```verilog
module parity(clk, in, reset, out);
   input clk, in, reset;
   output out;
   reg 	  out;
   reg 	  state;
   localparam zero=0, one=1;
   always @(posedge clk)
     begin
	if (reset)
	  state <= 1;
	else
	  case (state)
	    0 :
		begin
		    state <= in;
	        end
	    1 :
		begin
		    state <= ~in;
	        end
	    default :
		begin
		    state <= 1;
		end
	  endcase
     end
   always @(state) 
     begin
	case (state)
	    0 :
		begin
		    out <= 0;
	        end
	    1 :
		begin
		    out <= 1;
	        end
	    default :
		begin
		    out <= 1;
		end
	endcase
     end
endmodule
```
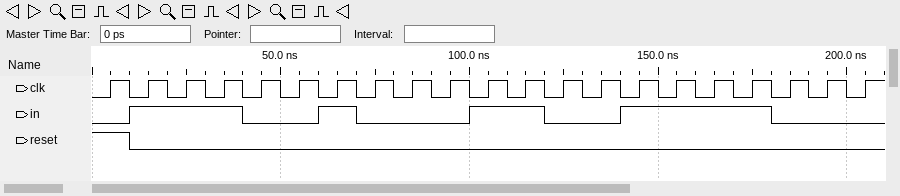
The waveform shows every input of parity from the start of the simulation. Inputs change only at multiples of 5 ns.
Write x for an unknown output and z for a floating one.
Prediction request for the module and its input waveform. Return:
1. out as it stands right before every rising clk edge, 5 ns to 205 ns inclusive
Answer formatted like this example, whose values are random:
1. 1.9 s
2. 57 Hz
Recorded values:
1. x 1 0 1 0 0 0 1 1 1 1 0 1 1 1 0 1 0 1 1 1
